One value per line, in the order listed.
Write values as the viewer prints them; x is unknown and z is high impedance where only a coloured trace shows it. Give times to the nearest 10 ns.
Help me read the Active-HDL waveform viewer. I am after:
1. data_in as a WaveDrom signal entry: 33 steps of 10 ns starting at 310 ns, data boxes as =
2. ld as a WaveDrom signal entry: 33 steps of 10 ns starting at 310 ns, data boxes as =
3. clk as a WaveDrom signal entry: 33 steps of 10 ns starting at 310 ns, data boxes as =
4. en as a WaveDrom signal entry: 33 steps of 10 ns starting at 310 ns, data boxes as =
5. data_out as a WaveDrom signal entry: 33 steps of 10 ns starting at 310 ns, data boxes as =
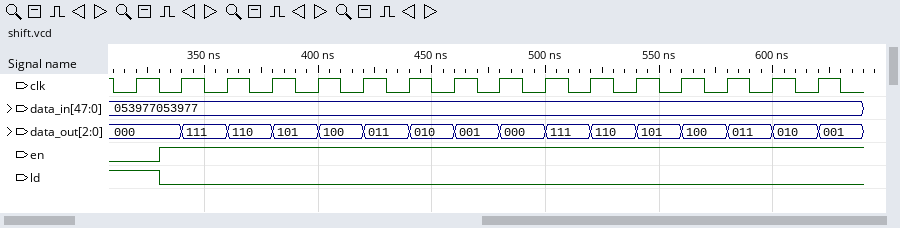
{name: 'data_in', wave: '=................................', data: '053977053977'}
{name: 'ld', wave: '1.0..............................'}
{name: 'clk', wave: '010101010101010101010101010101010'}
{name: 'en', wave: '0.1..............................'}
{name: 'data_out', wave: '=..=.=.=.=.=.=.=.=.=.=.=.=.=.=.=.', data: '000 111 110 101 100 011 010 001 000 111 110 101 100 011 010 001'}
